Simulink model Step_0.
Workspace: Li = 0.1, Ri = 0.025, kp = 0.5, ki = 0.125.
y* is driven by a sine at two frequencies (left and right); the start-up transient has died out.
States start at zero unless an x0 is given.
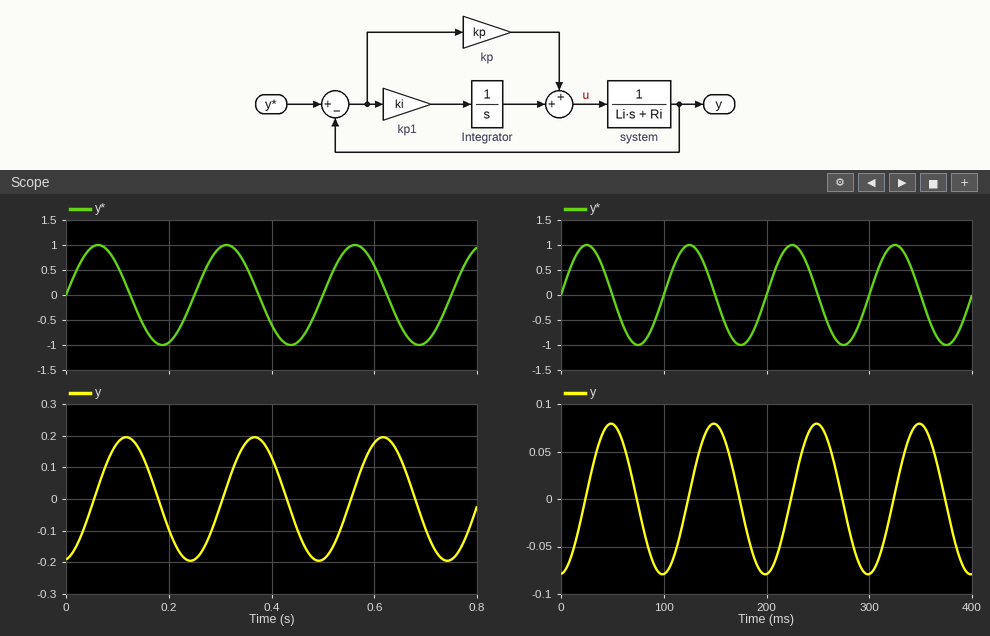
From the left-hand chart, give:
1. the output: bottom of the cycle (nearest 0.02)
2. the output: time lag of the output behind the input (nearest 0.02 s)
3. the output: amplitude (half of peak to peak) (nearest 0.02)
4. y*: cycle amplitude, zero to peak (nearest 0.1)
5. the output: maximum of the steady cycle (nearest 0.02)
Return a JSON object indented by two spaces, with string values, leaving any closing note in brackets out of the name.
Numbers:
{
  "the output: bottom of the cycle": "-0.20",
  "the output: time lag of the output behind the input": "0.06 s",
  "the output: amplitude (half of peak to peak)": "0.20",
  "y*: cycle amplitude, zero to peak": "1.0",
  "the output: maximum of the steady cycle": "0.20"
}
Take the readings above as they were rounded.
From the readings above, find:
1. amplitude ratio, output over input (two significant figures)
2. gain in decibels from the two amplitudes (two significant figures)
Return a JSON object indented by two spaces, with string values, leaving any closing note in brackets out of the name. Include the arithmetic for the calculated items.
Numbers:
{
  "amplitude ratio, output over input": "0.2 / 1 = 0.20",
  "gain in decibels from the two amplitudes": "20 log10(0.2 / 1) = -14 dB"
}
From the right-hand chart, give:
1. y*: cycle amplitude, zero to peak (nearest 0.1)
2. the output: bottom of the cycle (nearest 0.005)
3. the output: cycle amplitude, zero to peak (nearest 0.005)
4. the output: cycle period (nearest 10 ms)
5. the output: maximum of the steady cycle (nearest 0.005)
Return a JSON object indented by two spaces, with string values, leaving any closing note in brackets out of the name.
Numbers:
{
  "y*: cycle amplitude, zero to peak": "1.0",
  "the output: bottom of the cycle": "-0.080",
  "the output: cycle amplitude, zero to peak": "0.080",
  "the output: cycle period": "100 ms",
  "the output: maximum of the steady cycle": "0.080"
}
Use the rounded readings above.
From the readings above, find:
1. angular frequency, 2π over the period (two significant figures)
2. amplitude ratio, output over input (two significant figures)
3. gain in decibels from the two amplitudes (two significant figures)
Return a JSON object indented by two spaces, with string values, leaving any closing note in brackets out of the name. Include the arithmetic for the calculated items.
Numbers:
{
  "angular frequency, 2π over the period": "2π / 100 = 0.063 rad/ms",
  "amplitude ratio, output over input": "0.08 / 1 = 0.080",
  "gain in decibels from the two amplitudes": "20 log10(0.08 / 1) = -22 dB"
}
